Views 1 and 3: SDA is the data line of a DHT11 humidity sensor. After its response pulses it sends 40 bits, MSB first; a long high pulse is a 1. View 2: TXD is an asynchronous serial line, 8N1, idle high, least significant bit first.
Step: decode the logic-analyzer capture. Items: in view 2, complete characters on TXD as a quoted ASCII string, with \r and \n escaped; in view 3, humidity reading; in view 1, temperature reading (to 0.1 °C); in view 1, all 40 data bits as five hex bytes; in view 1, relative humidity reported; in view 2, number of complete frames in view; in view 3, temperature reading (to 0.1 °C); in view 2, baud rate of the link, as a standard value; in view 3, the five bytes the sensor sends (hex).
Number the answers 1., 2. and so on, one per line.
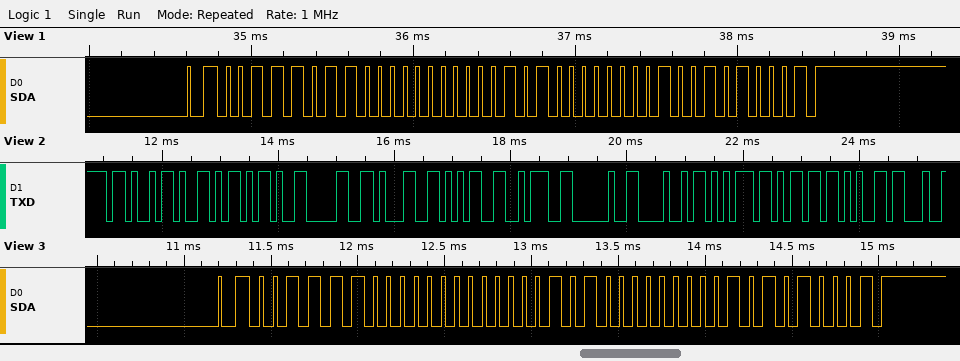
1. "KY-015: Hume"
2. 60 %
3. 20.2 °C
4. 3B 00 14 02 51
5. 59 %
6. 12
7. 20.1 °C
8. 9600 baud
9. 3C 00 14 01 51
